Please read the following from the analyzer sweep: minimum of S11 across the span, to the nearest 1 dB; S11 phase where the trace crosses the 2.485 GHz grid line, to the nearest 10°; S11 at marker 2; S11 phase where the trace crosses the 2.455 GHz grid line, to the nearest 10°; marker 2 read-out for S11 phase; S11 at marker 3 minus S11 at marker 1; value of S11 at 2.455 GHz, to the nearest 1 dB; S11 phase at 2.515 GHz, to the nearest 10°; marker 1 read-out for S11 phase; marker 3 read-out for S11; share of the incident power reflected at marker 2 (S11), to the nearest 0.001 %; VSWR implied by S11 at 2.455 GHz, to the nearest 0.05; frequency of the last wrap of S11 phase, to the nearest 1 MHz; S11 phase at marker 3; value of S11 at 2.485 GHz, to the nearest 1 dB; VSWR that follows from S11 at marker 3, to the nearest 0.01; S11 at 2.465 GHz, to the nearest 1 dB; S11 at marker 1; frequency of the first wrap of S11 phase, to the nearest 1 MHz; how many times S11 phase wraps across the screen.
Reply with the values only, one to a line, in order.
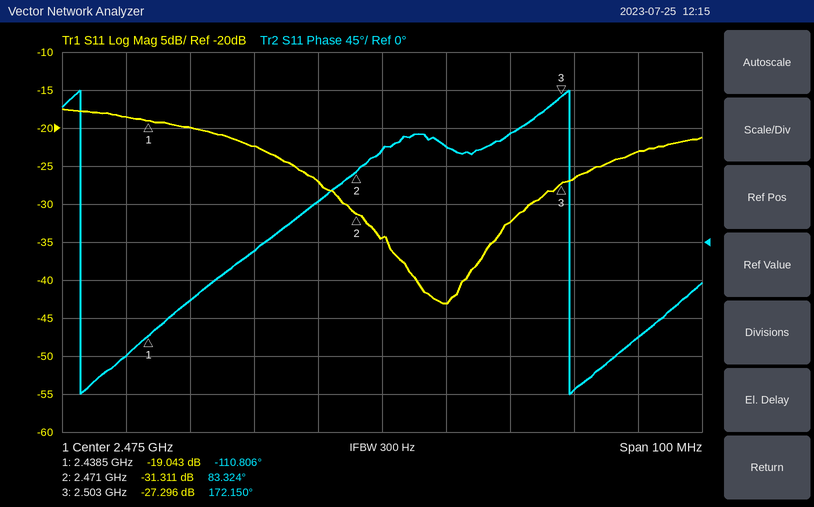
-43 dB
110°
-31.311 dB
-10°
83.324°
-8.253 dB
-22 dB
-110°
-110.806°
-27.296 dB
0.074 %
1.15
2.504 GHz
172.150°
-43 dB
1.09
-27 dB
-19.043 dB
2.428 GHz
2
